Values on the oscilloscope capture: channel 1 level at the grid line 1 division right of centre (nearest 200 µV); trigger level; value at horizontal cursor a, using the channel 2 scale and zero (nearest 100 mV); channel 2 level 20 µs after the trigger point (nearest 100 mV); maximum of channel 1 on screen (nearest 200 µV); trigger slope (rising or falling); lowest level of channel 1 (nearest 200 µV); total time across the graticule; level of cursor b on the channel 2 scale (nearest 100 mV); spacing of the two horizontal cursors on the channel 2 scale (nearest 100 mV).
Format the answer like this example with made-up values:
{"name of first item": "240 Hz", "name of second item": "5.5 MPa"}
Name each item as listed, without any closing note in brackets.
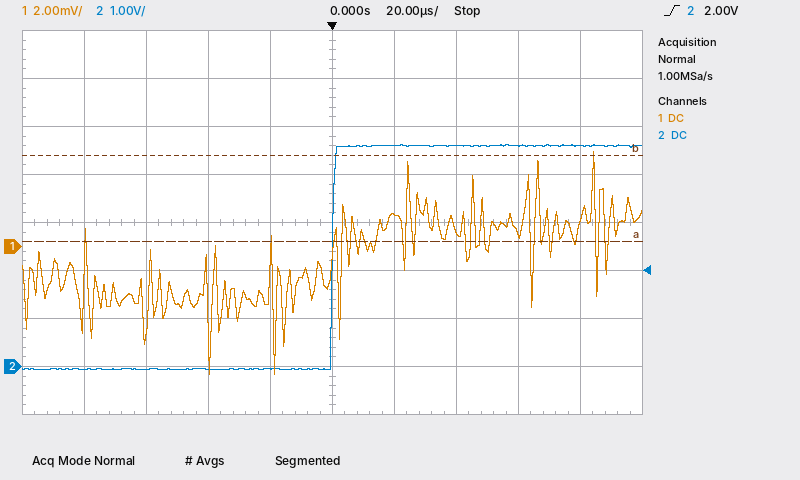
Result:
{"channel 1 level at the grid line 1 division right of centre": "1.4 mV", "trigger level": "2.00 V", "value at horizontal cursor a, using the channel 2 scale and zero": "2.6 V", "channel 2 level 20 µs after the trigger point": "4.6 V", "maximum of channel 1 on screen": "4.0 mV", "trigger slope": "rising", "lowest level of channel 1": "-5.4 mV", "total time across the graticule": "200 µs", "level of cursor b on the channel 2 scale": "4.4 V", "spacing of the two horizontal cursors on the channel 2 scale": "1.8 V"}
